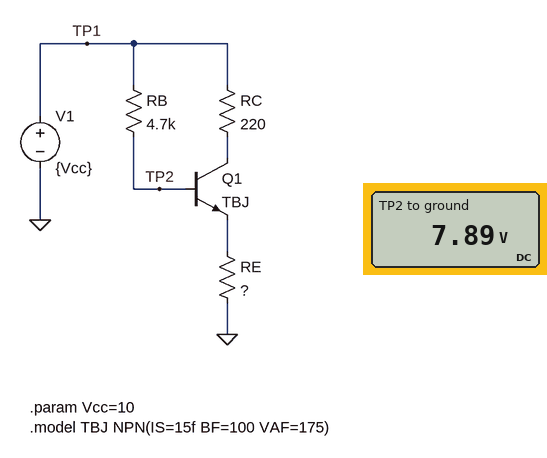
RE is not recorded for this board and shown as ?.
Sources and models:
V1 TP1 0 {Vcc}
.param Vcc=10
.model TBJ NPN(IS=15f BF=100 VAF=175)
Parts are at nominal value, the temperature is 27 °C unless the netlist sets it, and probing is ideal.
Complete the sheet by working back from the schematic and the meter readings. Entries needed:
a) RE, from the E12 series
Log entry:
560 Ω
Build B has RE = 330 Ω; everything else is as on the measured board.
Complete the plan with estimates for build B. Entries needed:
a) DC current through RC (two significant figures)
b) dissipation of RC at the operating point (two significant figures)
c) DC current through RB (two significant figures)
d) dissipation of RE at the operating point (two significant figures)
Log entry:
18 mA
68 mW
690 µA
110 mW
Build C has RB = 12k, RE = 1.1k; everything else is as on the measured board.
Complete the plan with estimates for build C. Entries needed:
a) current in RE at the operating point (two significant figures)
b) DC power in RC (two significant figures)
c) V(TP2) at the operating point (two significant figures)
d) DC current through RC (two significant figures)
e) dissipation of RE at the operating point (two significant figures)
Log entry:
7.5 mA
12 mW
8.9 V
7.4 mA
61 mW
